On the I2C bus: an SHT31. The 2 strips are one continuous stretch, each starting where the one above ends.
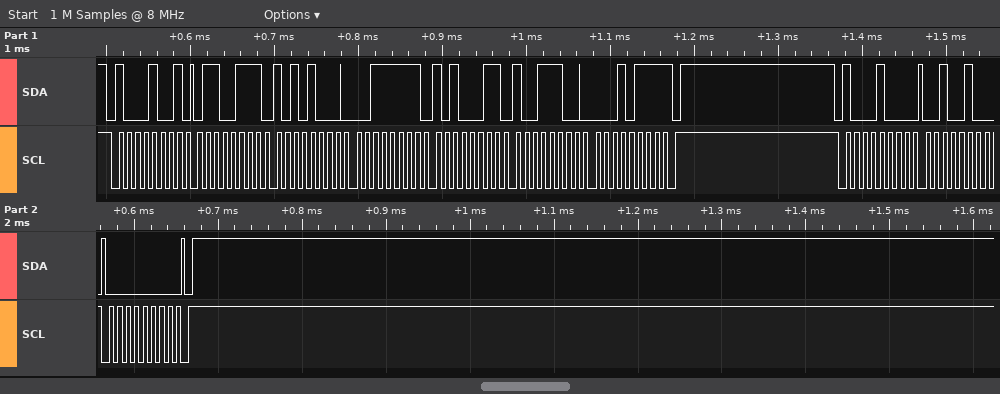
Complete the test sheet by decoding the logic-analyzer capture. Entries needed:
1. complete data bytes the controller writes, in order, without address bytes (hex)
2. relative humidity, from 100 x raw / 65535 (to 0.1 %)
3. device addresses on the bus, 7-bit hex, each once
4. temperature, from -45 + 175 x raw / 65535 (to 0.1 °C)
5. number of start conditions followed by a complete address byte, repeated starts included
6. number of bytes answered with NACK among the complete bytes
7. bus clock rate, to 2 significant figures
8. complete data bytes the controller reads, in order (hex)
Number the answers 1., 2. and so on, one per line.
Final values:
1. 24 00
2. 63.9 %
3. 0x44
4. 25.9 °C
5. 2
6. 1
7. 100 kHz
8. 67 A8 3F A3 9C 17
